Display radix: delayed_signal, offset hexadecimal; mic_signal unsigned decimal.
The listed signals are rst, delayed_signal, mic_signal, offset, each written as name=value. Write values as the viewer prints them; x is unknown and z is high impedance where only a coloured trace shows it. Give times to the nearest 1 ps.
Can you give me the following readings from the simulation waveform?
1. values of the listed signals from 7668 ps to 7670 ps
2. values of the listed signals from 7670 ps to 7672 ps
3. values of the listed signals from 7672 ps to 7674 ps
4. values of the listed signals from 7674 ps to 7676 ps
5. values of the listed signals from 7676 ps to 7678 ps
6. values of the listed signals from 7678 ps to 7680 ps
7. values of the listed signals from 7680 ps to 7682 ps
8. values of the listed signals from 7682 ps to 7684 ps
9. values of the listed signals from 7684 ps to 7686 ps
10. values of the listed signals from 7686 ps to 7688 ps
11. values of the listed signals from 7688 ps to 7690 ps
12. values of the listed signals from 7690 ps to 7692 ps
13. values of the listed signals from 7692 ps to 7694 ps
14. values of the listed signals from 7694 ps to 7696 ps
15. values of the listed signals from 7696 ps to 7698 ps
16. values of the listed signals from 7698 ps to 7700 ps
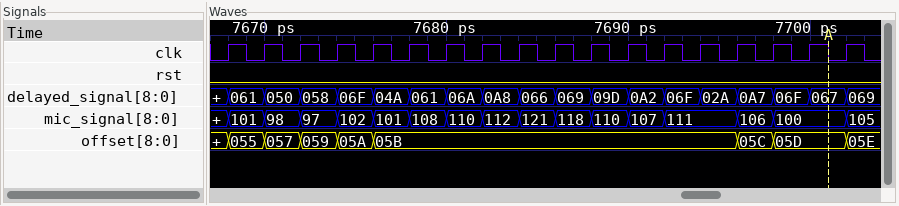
rst=0, delayed_signal=061, mic_signal=101, offset=055
rst=0, delayed_signal=050, mic_signal=98, offset=057
rst=0, delayed_signal=058, mic_signal=97, offset=059
rst=0, delayed_signal=06F, mic_signal=102, offset=05A
rst=0, delayed_signal=04A, mic_signal=101, offset=05B
rst=0, delayed_signal=061, mic_signal=108, offset=05B
rst=0, delayed_signal=06A, mic_signal=110, offset=05B
rst=0, delayed_signal=0A8, mic_signal=112, offset=05B
rst=0, delayed_signal=066, mic_signal=121, offset=05B
rst=0, delayed_signal=069, mic_signal=118, offset=05B
rst=0, delayed_signal=09D, mic_signal=110, offset=05B
rst=0, delayed_signal=0A2, mic_signal=107, offset=05B
rst=0, delayed_signal=06F, mic_signal=111, offset=05B
rst=0, delayed_signal=02A, mic_signal=111, offset=05B
rst=0, delayed_signal=0A7, mic_signal=106, offset=05C
rst=0, delayed_signal=06F, mic_signal=100, offset=05D
